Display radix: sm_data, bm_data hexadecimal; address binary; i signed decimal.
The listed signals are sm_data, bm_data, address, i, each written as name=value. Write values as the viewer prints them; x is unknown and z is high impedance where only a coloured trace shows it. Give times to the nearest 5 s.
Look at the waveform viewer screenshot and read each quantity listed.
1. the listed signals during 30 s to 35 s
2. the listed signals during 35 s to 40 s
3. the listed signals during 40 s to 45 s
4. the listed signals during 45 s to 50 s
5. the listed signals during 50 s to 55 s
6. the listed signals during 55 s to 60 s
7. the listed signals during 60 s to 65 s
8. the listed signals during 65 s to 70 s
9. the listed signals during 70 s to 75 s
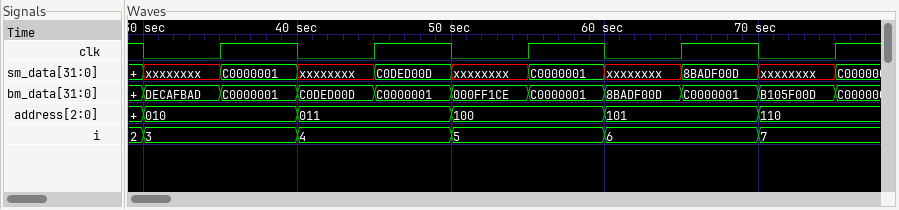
sm_data=xxxxxxxx, bm_data=DECAFBAD, address=010, i=3
sm_data=C0000001, bm_data=C0000001, address=010, i=3
sm_data=xxxxxxxx, bm_data=C0DED00D, address=011, i=4
sm_data=C0DED00D, bm_data=C0000001, address=011, i=4
sm_data=xxxxxxxx, bm_data=000FF1CE, address=100, i=5
sm_data=C0000001, bm_data=C0000001, address=100, i=5
sm_data=xxxxxxxx, bm_data=8BADF00D, address=101, i=6
sm_data=8BADF00D, bm_data=C0000001, address=101, i=6
sm_data=xxxxxxxx, bm_data=B105F00D, address=110, i=7
